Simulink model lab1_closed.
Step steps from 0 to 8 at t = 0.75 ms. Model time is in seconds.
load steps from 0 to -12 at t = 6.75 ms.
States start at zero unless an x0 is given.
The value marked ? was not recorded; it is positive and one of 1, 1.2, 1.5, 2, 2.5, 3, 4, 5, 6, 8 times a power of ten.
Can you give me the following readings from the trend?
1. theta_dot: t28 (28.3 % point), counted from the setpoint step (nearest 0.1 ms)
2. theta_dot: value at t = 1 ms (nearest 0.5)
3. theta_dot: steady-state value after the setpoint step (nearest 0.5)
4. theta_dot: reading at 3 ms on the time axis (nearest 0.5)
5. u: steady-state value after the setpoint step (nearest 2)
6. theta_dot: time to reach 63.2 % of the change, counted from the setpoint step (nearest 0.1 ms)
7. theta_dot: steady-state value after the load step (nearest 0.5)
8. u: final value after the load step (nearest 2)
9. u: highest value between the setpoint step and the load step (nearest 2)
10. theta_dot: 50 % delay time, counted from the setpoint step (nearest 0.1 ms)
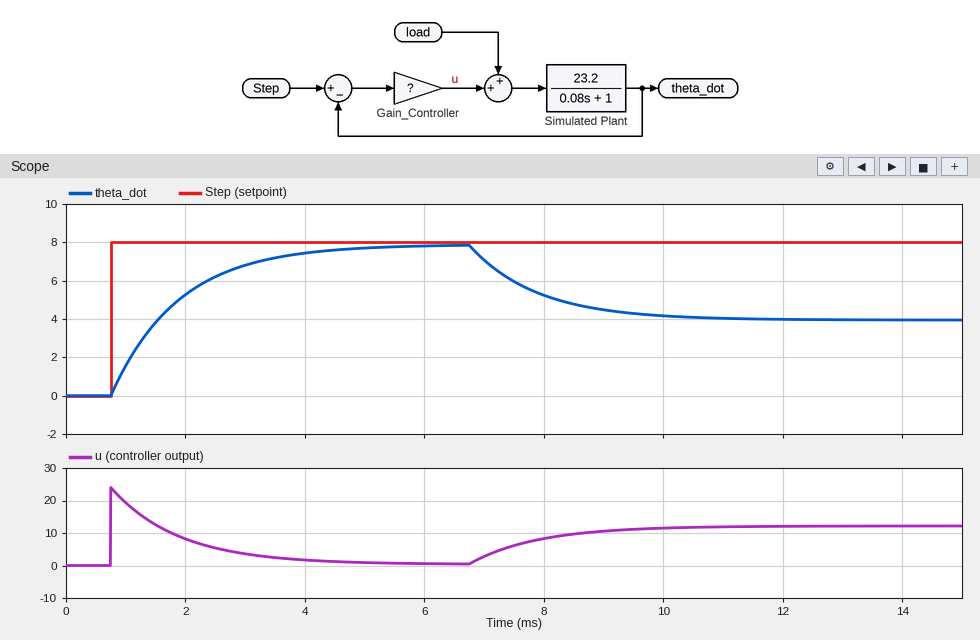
0.4 ms
1.5
8.0
7.0
0
1.1 ms
4.0
12
24
0.8 ms
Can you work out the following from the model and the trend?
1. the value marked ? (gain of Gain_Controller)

3
